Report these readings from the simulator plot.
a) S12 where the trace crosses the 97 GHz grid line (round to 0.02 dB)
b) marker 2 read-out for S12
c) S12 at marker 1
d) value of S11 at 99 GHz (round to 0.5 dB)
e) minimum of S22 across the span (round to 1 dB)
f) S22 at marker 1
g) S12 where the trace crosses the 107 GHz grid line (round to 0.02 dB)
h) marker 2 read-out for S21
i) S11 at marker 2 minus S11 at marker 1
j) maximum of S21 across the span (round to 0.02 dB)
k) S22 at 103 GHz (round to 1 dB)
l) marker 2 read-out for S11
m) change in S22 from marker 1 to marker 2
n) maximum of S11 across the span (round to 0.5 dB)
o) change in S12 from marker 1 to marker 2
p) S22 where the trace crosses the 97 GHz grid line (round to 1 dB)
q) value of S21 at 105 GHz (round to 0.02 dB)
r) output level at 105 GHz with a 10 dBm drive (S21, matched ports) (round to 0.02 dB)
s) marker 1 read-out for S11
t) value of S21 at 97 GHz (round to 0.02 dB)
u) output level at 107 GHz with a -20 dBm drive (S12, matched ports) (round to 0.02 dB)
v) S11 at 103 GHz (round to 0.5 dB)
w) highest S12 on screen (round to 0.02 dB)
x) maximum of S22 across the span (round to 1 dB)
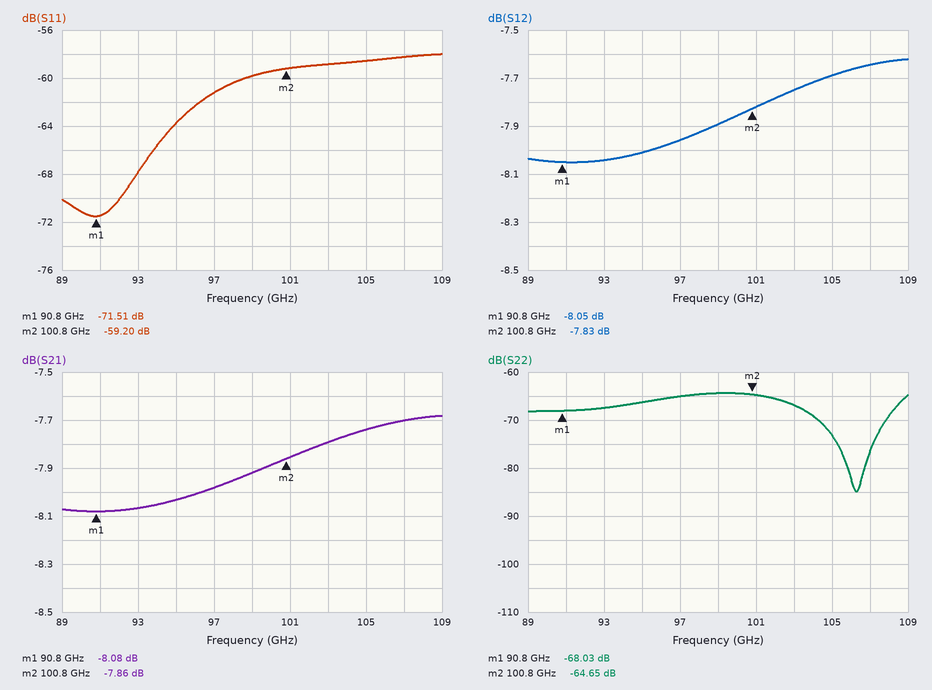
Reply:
-7.96 dB
-7.83 dB
-8.05 dB
-60.0 dB
-85 dB
-68.03 dB
-7.64 dB
-7.86 dB
12.31 dB
-7.68 dB
-67 dB
-59.20 dB
3.38 dB
-58.0 dB
0.22 dB
-65 dB
-7.74 dB
2.26 dBm
-71.51 dB
-7.98 dB
-27.64 dBm
-59.0 dB
-7.62 dB
-64 dB
